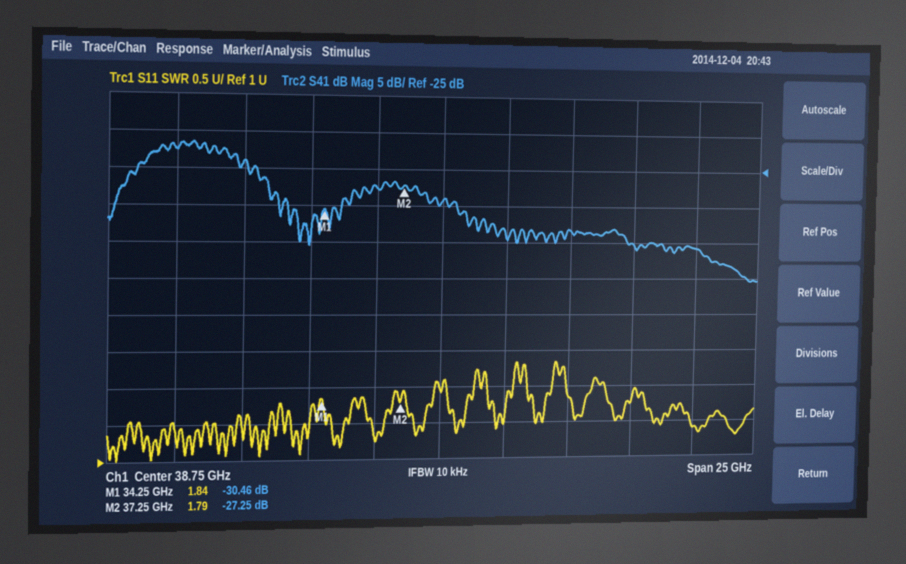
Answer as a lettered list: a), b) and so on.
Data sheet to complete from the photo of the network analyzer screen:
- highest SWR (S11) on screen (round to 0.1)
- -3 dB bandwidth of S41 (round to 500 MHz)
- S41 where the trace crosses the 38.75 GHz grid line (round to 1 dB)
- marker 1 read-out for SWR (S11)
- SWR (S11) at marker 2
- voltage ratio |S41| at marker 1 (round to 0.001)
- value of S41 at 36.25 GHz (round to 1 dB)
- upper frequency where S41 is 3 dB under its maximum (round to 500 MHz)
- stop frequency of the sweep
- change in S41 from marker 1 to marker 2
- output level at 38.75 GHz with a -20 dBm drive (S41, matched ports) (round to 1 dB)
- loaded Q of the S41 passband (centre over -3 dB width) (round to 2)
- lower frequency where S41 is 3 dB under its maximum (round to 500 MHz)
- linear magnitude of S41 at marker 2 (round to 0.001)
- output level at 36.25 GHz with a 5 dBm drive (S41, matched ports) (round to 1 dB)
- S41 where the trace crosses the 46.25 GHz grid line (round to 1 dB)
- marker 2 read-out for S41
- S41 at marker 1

a) 2.3
b) 3.5 GHz
c) -29 dB
d) 1.84
e) 1.79
f) 0.030
g) -28 dB
h) 31.0 GHz
i) 51.25 GHz
j) 3.21 dB
k) -49 dBm
l) 8
m) 27.5 GHz
n) 0.043
o) -23 dBm
p) -35 dB
q) -27.25 dB
r) -30.46 dB
